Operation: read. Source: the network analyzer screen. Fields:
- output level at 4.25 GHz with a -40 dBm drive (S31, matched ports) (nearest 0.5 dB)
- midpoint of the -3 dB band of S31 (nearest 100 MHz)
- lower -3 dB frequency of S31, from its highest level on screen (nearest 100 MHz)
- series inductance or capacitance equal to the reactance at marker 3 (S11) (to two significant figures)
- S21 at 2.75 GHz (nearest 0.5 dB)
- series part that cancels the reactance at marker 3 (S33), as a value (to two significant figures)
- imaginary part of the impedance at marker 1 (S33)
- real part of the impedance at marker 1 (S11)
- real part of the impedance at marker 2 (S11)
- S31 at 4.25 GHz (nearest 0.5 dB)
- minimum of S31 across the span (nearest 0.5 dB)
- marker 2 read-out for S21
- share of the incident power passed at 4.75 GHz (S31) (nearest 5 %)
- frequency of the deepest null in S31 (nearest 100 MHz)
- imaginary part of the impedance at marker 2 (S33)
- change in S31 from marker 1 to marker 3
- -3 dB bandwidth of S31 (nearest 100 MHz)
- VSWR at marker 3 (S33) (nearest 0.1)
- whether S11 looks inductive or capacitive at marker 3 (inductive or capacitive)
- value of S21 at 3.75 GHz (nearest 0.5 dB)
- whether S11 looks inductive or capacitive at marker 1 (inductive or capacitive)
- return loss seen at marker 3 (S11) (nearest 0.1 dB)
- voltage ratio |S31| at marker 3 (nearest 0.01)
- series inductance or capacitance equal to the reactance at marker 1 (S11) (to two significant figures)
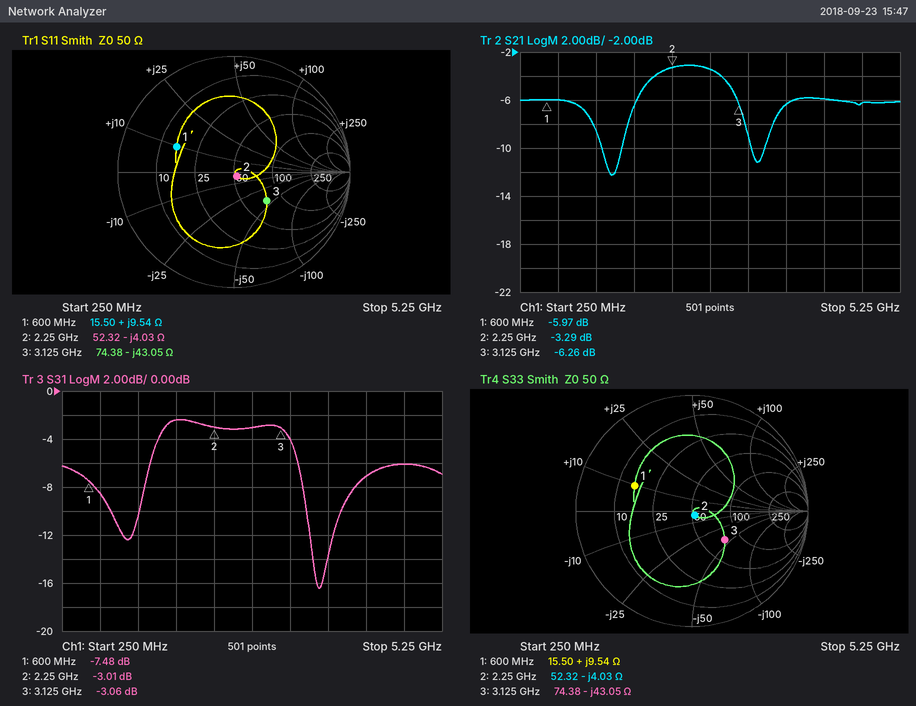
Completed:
-47.0 dBm
2.4 GHz
1.4 GHz
1.2 pF
-3.5 dB
2.2 nH
+9.54 Ω
15.50 Ω
52.32 Ω
-7.0 dB
-16.5 dB
-3.29 dB
25 %
3.6 GHz
-4.03 Ω
4.42 dB
1.9 GHz
2.2
capacitive
-6.5 dB
inductive
8.5 dB
0.70
2.5 nH
